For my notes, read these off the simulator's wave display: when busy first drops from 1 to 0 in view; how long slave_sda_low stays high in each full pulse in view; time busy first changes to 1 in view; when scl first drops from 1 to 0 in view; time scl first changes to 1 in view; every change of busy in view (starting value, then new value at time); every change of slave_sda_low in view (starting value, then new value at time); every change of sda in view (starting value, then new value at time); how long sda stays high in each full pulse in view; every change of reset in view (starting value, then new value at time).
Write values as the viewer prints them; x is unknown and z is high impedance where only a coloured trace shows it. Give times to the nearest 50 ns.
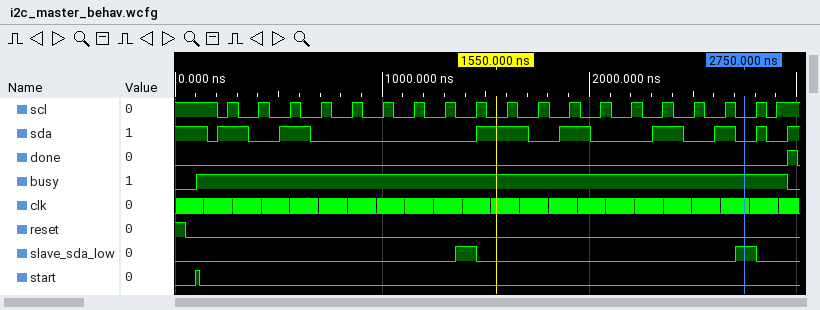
2950 ns
100 ns, 100 ns
100 ns
200 ns
250 ns
0, 1 at 100 ns, 0 at 2950 ns
0, 1 at 1350 ns, 0 at 1450 ns, 1 at 2700 ns, 0 at 2800 ns
1, 0 at 150 ns, 1 at 200 ns, 0 at 350 ns, 1 at 500 ns, 0 at 650 ns, 1 at 1450 ns, 0 at 1700 ns, 1 at 1850 ns, 0 at 2000 ns, 1 at 2300 ns, 0 at 2450 ns, 1 at 2600 ns, 0 at 2700 ns, 1 at 2800 ns, 0 at 2850 ns, 1 at 2950 ns
150 ns, 150 ns, 250 ns, 150 ns, 150 ns, 100 ns, 50 ns
1, 0 at 50 ns
